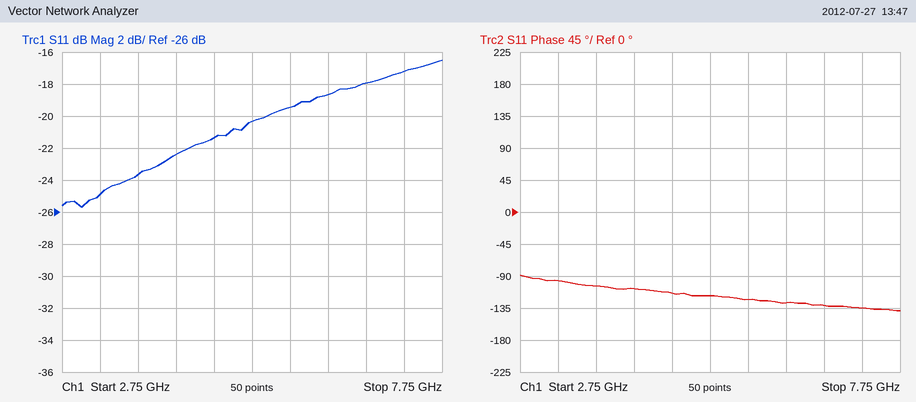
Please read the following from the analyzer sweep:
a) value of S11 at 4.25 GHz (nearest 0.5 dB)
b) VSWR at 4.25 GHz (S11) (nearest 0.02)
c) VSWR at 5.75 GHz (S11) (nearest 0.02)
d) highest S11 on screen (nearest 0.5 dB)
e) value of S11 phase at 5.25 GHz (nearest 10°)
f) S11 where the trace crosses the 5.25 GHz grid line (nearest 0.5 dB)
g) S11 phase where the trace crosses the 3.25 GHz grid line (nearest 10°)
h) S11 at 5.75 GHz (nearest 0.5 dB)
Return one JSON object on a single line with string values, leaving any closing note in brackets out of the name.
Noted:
{"value of S11 at 4.25 GHz": "-22.5 dB", "VSWR at 4.25 GHz (S11)": "1.16", "VSWR at 5.75 GHz (S11)": "1.24", "highest S11 on screen": "-16.5 dB", "value of S11 phase at 5.25 GHz": "-120°", "S11 where the trace crosses the 5.25 GHz grid line": "-20.5 dB", "S11 phase where the trace crosses the 3.25 GHz grid line": "-100°", "S11 at 5.75 GHz": "-19.5 dB"}
